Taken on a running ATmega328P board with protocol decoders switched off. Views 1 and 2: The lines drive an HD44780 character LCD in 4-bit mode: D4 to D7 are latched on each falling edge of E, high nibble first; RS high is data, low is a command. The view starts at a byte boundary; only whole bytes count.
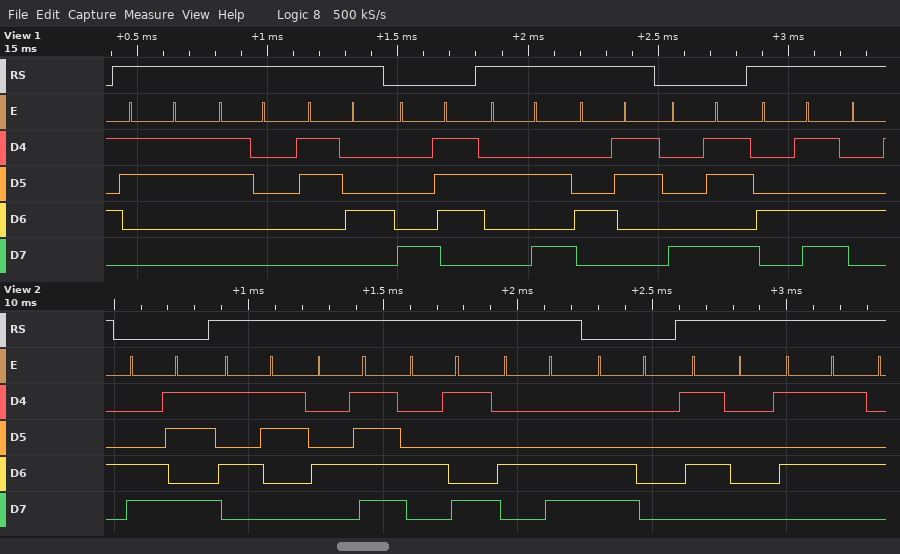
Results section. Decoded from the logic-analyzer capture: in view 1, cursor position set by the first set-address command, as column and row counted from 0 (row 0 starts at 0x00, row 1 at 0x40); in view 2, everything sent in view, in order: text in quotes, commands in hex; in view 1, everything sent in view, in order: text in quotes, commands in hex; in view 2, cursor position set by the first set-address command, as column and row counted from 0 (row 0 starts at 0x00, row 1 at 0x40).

column 7, row 0
0xCB "SOIL" 0xC0 "PU"
"304" 0x87 "*C" 0x8B "M"
column 11, row 1
